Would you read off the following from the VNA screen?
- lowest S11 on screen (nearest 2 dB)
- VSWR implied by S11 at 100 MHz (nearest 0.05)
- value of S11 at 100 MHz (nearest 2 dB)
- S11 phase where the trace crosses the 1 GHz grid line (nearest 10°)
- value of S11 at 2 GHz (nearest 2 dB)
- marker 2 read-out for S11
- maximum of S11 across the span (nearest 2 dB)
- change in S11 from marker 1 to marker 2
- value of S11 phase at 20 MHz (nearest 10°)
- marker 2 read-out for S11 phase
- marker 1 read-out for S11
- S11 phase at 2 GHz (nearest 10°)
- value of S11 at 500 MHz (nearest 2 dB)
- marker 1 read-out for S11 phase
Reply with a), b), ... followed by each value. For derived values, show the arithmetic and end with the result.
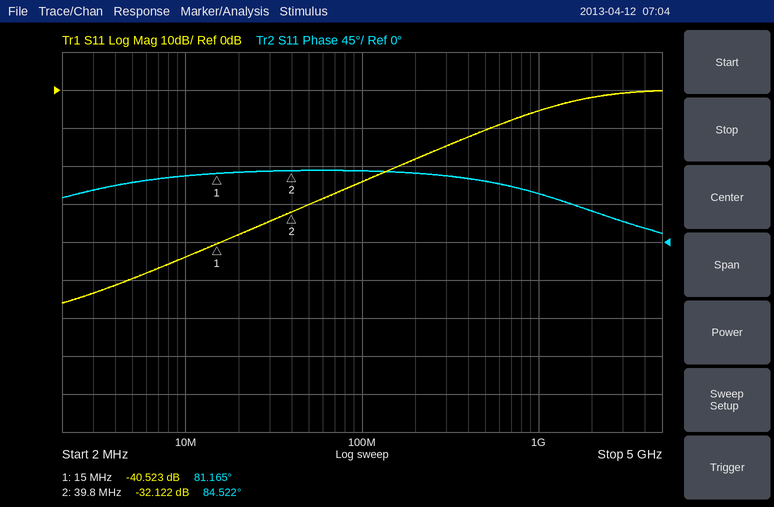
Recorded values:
a) -56 dB
b) |Γ| = 10^(-24/20) = 0.0631; VSWR = (1 + 0.0631)/(1 − 0.0631) ≈ 1.13, so 1.15 to the nearest 0.05
c) -24 dB
d) 60°
e) -2 dB
f) -32.122 dB
g) 0 dB
h) -32.122 − (-40.523) = 8.401 dB
i) 80°
j) 84.522°
k) -40.523 dB
l) 40°
m) -10 dB
n) 81.165°
